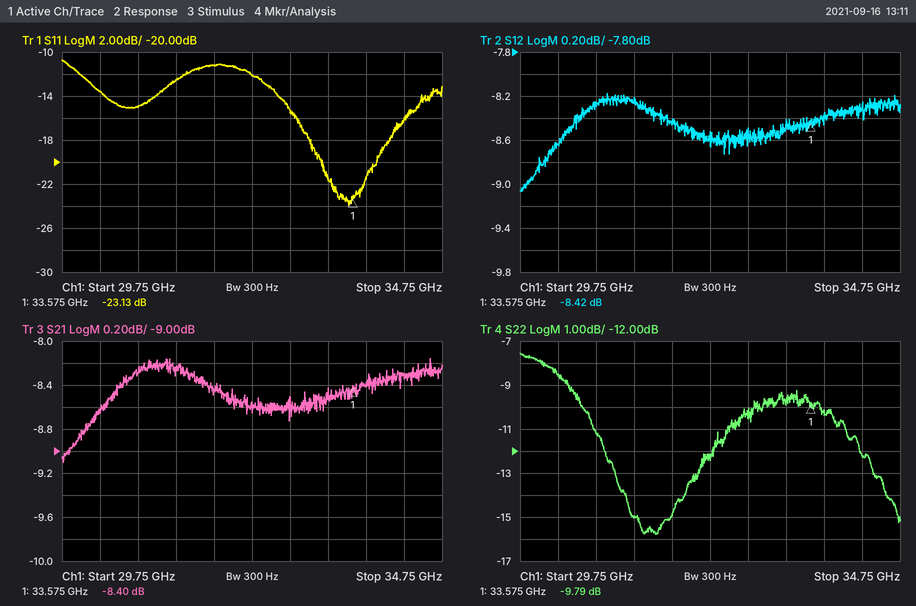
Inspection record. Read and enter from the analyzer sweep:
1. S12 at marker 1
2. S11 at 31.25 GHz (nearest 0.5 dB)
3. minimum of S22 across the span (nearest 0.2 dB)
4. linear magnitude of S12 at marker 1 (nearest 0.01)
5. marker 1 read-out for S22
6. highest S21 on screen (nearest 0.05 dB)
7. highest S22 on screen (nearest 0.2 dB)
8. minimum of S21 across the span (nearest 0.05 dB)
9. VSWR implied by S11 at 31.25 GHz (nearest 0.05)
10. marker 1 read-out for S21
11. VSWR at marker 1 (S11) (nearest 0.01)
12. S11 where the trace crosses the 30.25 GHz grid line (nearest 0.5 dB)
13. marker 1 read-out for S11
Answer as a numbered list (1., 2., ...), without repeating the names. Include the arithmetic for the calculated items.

1. -8.42 dB
2. -12.5 dB
3. -15.8 dB
4. 10^(-8.42/20) ≈ 0.38
5. -9.79 dB
6. -8.15 dB
7. -7.6 dB
8. -9.10 dB
9. |Γ| = 10^(-12.5/20) = 0.2371; VSWR = (1 + 0.2371)/(1 − 0.2371) ≈ 1.62, so 1.60 to the nearest 0.05
10. -8.40 dB
11. (1 + 0.0697)/(1 − 0.0697) ≈ 1.15
12. -13.5 dB
13. -23.13 dB
